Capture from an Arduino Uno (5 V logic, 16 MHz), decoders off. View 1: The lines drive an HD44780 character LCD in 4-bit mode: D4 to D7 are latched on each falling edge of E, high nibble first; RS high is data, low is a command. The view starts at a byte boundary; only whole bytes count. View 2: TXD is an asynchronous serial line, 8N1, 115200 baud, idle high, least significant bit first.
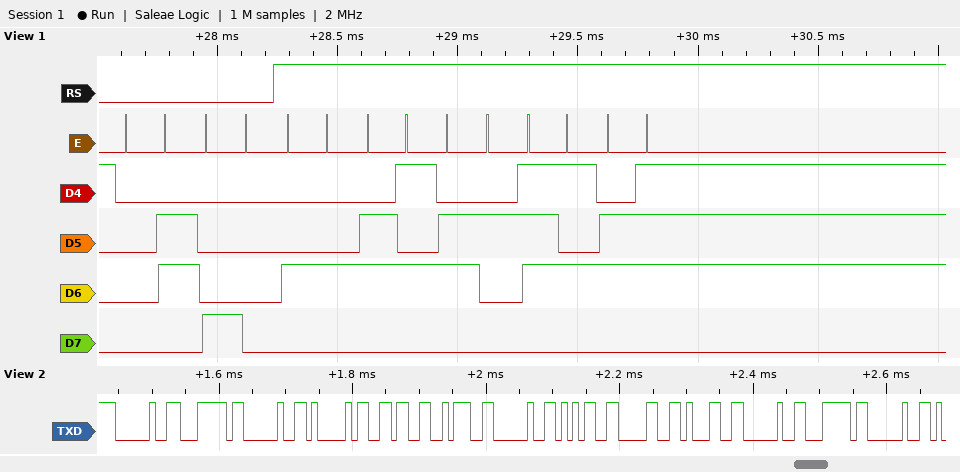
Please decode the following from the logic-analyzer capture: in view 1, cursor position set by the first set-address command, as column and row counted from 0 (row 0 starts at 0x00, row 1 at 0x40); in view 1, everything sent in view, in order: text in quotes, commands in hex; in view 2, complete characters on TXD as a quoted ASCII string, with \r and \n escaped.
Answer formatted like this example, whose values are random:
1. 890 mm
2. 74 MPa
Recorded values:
1. column 0, row 0
2. 0x06 0x80 "Debug"
3. " | A6: 501 | "
